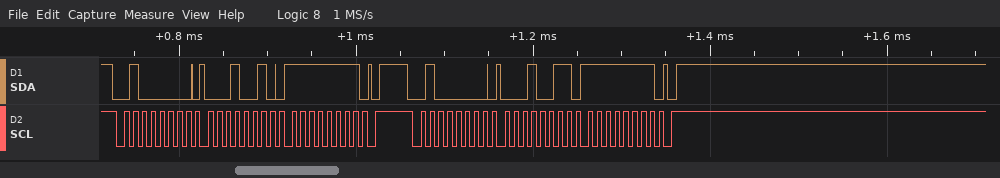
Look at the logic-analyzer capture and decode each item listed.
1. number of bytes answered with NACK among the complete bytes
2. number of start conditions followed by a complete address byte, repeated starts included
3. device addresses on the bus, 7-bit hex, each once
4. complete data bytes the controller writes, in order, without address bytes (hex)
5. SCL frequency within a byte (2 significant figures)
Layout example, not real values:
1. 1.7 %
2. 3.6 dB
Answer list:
1. 0
2. 2
3. 0x20
4. 12 FF 13 FF
5. 100 kHz
